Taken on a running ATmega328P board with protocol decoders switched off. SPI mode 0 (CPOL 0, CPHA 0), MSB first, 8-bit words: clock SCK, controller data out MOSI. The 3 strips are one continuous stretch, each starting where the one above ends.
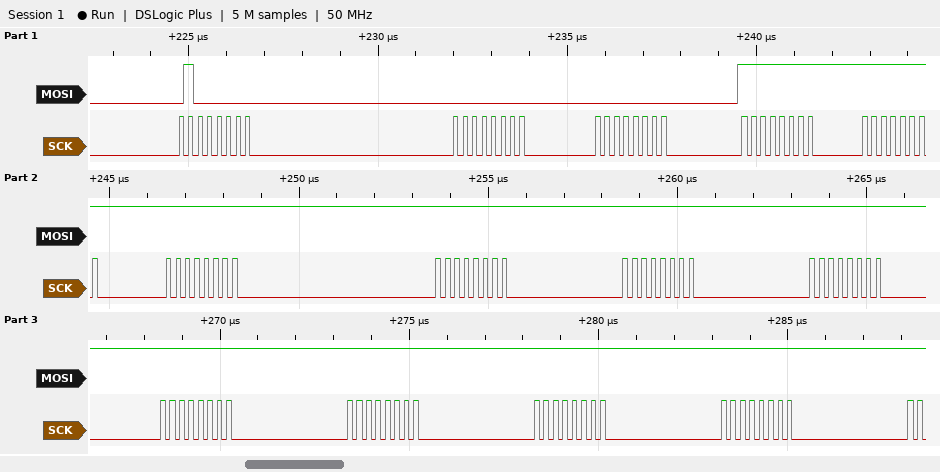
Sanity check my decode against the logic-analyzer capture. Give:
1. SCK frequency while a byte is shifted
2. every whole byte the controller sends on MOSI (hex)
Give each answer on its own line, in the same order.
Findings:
4 MHz
40 00 00 FF FF FF FF FF FF FF FF FF FF
